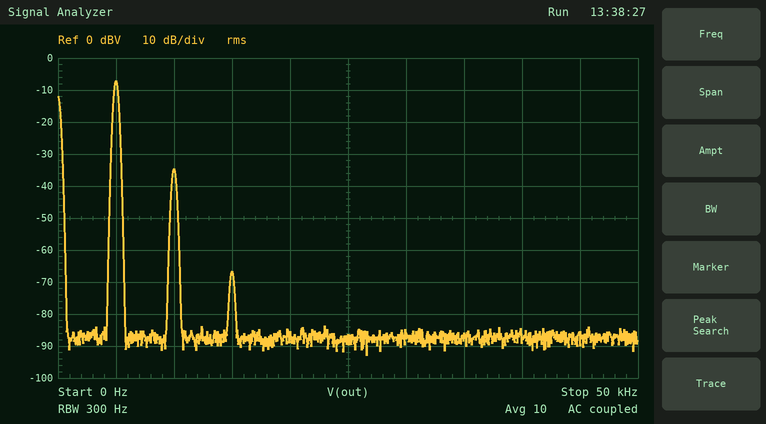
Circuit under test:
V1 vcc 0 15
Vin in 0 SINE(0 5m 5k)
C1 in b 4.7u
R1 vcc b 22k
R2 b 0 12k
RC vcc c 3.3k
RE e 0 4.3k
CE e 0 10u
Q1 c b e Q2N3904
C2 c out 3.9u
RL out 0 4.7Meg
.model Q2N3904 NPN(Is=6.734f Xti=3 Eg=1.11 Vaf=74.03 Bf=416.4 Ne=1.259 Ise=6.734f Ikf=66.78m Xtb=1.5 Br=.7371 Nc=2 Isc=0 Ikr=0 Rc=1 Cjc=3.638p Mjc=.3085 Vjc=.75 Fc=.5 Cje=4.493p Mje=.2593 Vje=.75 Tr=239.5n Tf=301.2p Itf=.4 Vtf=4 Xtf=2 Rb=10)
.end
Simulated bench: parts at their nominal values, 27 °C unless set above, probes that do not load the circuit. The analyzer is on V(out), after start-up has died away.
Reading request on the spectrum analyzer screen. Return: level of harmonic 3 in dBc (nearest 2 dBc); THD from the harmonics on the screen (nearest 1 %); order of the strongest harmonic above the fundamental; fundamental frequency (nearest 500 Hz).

-60 dBc
4 %
2
5.0 kHz
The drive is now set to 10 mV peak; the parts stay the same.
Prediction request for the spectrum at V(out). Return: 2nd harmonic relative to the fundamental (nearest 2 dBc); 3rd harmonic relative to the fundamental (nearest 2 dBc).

-22 dBc
-48 dBc
